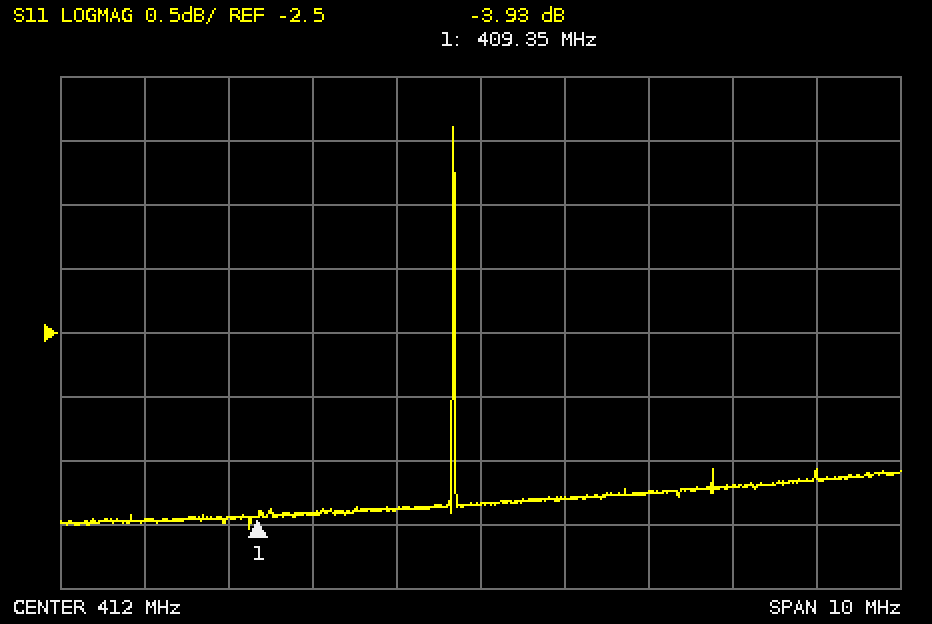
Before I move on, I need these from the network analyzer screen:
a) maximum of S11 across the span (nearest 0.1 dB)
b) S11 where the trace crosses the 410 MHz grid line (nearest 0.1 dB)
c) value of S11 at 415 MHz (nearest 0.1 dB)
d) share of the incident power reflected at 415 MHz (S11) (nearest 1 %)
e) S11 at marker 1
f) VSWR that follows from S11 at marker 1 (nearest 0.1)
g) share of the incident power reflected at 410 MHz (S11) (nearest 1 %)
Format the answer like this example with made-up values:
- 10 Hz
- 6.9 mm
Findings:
- -0.9 dB
- -3.9 dB
- -3.7 dB
- 43 %
- -3.93 dB
- 4.5
- 41 %
